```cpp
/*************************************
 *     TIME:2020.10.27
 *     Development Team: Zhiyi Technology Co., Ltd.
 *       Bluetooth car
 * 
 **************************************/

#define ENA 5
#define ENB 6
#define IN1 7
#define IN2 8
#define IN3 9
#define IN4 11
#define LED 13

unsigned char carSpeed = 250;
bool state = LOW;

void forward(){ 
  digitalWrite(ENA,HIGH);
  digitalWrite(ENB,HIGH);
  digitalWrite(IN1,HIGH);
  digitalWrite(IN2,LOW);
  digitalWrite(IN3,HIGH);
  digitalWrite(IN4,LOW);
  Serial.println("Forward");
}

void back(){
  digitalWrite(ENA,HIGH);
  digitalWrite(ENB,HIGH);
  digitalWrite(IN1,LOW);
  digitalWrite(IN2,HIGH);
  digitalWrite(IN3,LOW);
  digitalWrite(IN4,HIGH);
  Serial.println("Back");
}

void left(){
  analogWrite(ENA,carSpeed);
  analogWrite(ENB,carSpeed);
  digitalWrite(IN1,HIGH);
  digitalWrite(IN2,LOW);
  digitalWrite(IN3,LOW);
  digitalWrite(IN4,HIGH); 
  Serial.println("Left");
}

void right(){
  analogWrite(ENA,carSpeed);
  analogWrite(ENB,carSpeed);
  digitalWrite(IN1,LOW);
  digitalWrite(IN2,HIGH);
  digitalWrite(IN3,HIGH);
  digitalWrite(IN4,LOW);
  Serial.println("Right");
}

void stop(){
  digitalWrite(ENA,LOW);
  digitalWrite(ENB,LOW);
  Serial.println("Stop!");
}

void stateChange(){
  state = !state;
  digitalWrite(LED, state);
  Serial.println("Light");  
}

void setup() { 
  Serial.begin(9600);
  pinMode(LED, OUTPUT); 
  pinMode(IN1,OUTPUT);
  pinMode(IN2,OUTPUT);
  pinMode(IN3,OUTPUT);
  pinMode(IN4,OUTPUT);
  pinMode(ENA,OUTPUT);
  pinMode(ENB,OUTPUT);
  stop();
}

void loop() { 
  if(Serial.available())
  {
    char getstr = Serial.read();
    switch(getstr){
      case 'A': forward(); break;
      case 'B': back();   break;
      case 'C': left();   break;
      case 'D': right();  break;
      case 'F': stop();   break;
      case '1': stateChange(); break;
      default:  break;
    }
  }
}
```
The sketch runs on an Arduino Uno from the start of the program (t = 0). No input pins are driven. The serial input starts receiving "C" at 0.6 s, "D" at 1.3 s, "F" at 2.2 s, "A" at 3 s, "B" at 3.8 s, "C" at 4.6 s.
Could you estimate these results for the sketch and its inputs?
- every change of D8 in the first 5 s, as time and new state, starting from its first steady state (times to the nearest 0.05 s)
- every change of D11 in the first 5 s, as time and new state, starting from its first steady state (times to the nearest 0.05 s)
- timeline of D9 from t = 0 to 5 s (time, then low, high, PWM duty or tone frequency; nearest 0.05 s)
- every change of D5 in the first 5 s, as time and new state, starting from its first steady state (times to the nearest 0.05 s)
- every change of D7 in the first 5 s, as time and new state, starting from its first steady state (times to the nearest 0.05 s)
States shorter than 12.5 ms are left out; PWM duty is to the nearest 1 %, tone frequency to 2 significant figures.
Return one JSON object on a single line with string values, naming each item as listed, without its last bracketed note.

{"every change of D8 in the first 5 s, as time and new state, starting from its first steady state": "0 s low; 1.3 s high; 3 s low; 3.8 s high; 4.6 s low", "every change of D11 in the first 5 s, as time and new state, starting from its first steady state": "0 s low; 0.6 s high; 1.3 s low; 3.8 s high", "timeline of D9 from t = 0 to 5 s": "0 s low; 1.3 s high; 3.8 s low", "every change of D5 in the first 5 s, as time and new state, starting from its first steady state": "0 s low; 0.6 s PWM 98 %; 2.2 s low; 3 s high; 4.6 s PWM 98 %", "every change of D7 in the first 5 s, as time and new state, starting from its first steady state": "0 s low; 0.6 s high; 1.3 s low; 3 s high; 3.8 s low; 4.6 s high"}
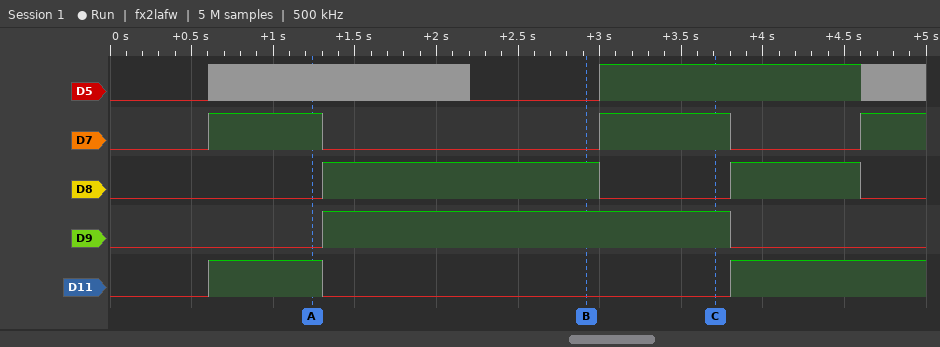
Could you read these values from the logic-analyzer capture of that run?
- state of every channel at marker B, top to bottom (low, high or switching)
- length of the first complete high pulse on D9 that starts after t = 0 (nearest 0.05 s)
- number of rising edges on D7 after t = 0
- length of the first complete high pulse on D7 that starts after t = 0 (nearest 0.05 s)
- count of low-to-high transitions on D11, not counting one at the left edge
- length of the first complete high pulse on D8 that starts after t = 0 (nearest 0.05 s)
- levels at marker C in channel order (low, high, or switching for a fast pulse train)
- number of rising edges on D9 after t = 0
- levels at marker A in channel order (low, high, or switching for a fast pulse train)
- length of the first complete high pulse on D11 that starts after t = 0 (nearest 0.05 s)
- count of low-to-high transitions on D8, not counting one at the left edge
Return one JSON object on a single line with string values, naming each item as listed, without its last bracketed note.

{"state of every channel at marker B, top to bottom": "D5 low, D7 low, D8 high, D9 high, D11 low", "length of the first complete high pulse on D9 that starts after t = 0": "2.50 s", "number of rising edges on D7 after t = 0": "3", "length of the first complete high pulse on D7 that starts after t = 0": "0.70 s", "count of low-to-high transitions on D11, not counting one at the left edge": "2", "length of the first complete high pulse on D8 that starts after t = 0": "1.70 s", "levels at marker C in channel order": "D5 high, D7 high, D8 low, D9 high, D11 low", "number of rising edges on D9 after t = 0": "1", "levels at marker A in channel order": "D5 switching, D7 high, D8 low, D9 low, D11 high", "length of the first complete high pulse on D11 that starts after t = 0": "0.70 s", "count of low-to-high transitions on D8, not counting one at the left edge": "2"}
